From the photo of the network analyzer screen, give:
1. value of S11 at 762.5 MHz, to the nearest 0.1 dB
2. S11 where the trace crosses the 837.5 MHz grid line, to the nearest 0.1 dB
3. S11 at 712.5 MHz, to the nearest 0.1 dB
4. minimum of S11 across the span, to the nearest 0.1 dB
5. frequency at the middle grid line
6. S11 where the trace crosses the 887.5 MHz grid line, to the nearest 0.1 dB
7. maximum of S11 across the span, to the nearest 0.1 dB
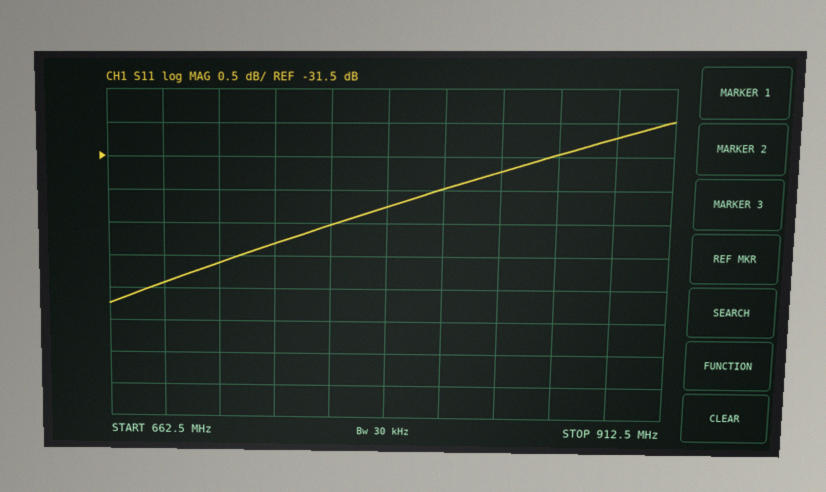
-32.5 dB
-31.7 dB
-33.1 dB
-33.7 dB
787.5 MHz
-31.2 dB
-31.0 dB
